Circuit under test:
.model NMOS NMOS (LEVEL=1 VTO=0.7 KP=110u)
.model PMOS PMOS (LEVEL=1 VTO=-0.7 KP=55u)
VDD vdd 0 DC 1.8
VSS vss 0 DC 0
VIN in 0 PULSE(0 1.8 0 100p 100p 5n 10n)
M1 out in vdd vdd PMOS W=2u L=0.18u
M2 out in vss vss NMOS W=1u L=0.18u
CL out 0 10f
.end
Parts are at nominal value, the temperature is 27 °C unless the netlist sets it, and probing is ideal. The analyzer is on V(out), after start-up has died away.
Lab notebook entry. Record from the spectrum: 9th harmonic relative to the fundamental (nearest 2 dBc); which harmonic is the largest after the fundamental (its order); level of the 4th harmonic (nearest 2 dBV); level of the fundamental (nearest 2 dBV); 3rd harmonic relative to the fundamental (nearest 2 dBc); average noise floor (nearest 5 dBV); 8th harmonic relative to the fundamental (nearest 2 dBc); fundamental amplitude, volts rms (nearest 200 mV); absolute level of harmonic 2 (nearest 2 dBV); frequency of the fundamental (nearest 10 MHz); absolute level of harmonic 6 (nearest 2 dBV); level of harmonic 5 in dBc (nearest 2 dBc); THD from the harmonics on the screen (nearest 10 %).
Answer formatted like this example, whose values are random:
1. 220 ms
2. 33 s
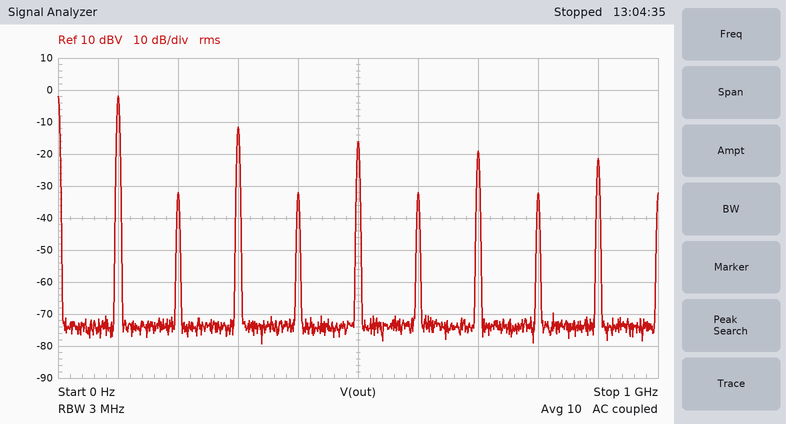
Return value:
1. -20 dBc
2. 3
3. -32 dBV
4. -2 dBV
5. -10 dBc
6. -75 dBV
7. -30 dBc
8. 800 mV
9. -32 dBV
10. 100 MHz
11. -32 dBV
12. -14 dBc
13. 40 %
